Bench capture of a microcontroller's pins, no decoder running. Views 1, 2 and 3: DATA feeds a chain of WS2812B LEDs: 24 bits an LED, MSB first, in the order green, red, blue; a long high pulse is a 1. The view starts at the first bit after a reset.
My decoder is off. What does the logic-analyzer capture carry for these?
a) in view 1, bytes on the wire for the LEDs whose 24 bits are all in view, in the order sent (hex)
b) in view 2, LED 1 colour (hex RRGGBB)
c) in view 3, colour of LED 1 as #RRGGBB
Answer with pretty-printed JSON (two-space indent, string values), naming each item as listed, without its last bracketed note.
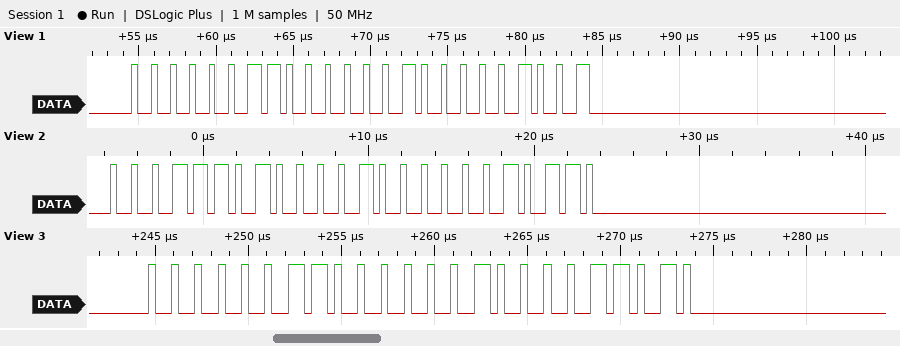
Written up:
{
  "in view 1, bytes on the wire for the LEDs whose 24 bits are all in view, in the order sent": "03 02 09",
  "in view 2, LED 1 colour": "#081D16",
  "in view 3, colour of LED 1 as #RRGGBB": "#02031A"
}
